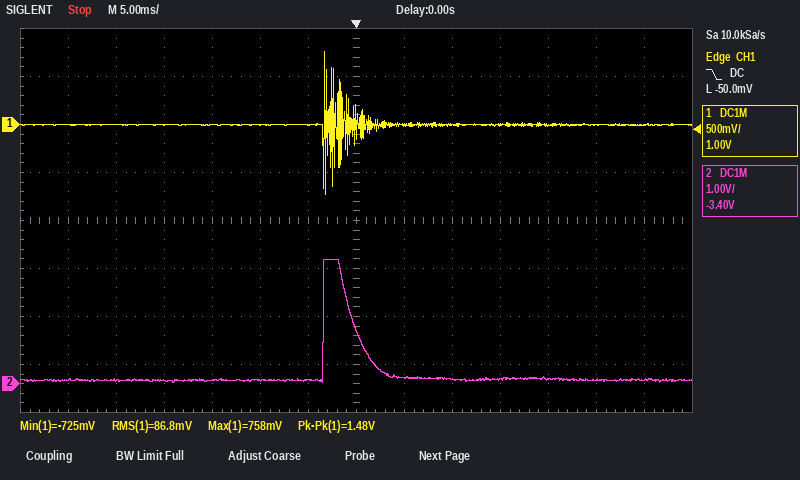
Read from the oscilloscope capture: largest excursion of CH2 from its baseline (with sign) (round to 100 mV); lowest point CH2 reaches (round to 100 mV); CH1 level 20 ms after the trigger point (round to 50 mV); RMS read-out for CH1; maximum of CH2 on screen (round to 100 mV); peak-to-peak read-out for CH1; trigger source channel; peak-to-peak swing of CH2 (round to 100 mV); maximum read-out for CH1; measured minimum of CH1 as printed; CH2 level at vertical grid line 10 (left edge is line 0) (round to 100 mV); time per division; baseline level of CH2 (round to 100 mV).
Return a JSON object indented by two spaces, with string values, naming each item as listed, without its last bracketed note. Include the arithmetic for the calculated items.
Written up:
{
  "largest excursion of CH2 from its baseline (with sign)": "2.6 V − (100 mV) = +2.5 V",
  "lowest point CH2 reaches": "0.0 V",
  "CH1 level 20 ms after the trigger point": "0 mV",
  "RMS read-out for CH1": "86.8 mV",
  "maximum of CH2 on screen": "2.6 V",
  "peak-to-peak read-out for CH1": "1.48 V",
  "trigger source channel": "CH1",
  "peak-to-peak swing of CH2": "2.6 V − (0.0 V) = 2.6 V",
  "maximum read-out for CH1": "758 mV",
  "measured minimum of CH1 as printed": "-725 mV",
  "CH2 level at vertical grid line 10 (left edge is line 0)": "100 mV",
  "time per division": "5 ms",
  "baseline level of CH2": "100 mV"
}
